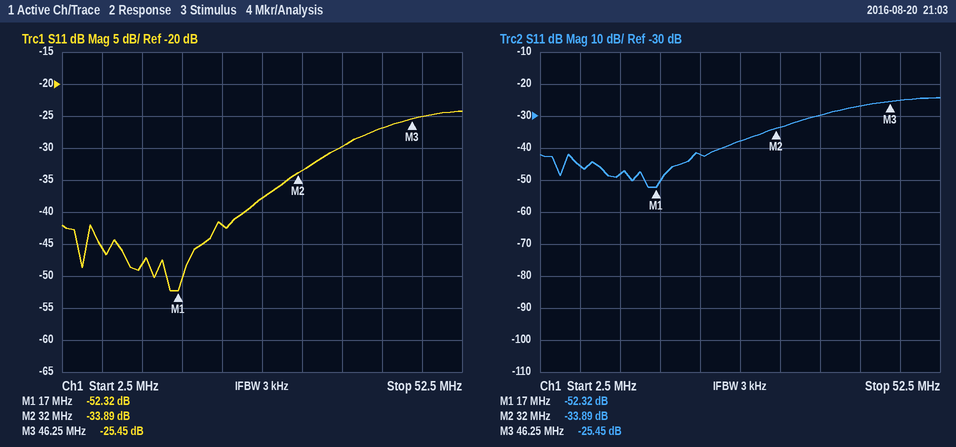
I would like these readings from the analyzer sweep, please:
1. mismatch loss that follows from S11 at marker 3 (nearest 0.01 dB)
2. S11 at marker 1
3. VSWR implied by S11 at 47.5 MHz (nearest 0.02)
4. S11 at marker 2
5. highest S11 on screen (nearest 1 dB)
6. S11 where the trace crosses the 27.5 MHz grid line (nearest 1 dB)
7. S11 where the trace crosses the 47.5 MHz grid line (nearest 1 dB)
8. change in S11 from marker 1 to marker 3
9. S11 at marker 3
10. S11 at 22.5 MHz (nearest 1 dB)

0.01 dB
-52.32 dB
1.12
-33.89 dB
-24 dB
-38 dB
-25 dB
26.87 dB
-25.45 dB
-42 dB
